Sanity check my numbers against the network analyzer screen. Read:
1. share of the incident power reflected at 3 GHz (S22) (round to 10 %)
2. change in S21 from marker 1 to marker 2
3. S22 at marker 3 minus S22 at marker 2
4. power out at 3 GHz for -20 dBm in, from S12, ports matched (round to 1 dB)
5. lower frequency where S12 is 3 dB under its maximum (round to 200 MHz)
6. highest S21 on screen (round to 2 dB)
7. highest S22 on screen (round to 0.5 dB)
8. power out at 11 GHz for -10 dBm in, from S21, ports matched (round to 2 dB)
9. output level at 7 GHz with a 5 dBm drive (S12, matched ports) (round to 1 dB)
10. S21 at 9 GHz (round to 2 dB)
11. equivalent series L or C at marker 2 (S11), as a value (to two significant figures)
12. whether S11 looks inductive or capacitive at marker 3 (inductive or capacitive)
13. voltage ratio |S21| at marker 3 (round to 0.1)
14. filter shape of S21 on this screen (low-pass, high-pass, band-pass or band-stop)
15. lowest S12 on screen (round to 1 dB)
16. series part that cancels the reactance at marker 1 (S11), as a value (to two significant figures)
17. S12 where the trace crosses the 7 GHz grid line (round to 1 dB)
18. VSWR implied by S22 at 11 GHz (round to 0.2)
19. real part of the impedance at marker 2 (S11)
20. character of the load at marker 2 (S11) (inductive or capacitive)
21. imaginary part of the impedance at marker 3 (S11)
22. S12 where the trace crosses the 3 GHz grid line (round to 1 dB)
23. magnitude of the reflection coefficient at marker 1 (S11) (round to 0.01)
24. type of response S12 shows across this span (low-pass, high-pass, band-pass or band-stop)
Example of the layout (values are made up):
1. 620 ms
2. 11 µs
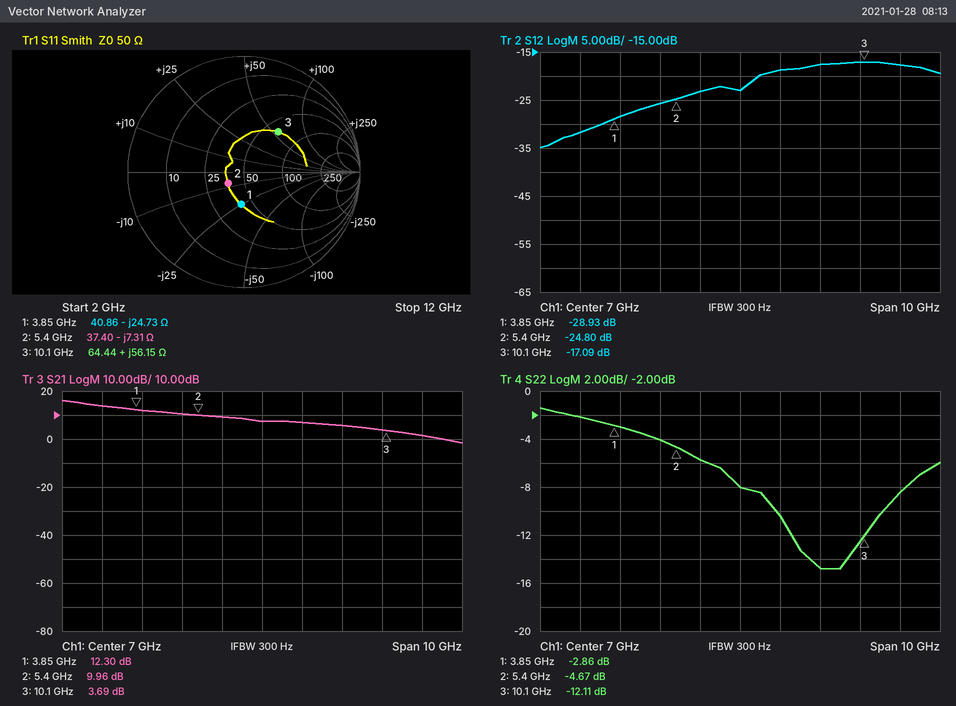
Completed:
1. 60 %
2. -2.34 dB
3. -7.44 dB
4. -52 dBm
5. 7.4 GHz
6. 16 dB
7. -1.5 dB
8. -8 dBm
9. -18 dBm
10. 6 dB
11. 4.0 pF
12. inductive
13. 1.5
14. low-pass
15. -35 dB
16. 1.0 nH
17. -23 dB
18. 2.2
19. 37.40 Ω
20. capacitive
21. +56.15 Ω
22. -32 dB
23. 0.28
24. high-pass
